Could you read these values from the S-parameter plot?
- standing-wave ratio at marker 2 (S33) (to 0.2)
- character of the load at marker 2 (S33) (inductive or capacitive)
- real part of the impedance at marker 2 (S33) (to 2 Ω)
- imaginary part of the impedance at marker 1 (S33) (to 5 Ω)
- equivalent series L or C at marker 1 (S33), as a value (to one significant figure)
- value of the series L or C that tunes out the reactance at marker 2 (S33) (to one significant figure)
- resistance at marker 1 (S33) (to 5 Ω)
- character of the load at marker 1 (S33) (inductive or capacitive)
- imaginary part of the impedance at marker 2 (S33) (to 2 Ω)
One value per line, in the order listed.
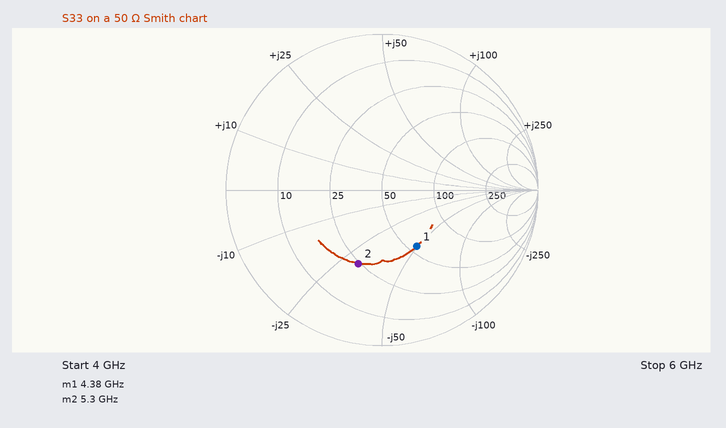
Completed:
3.0
capacitive
24 Ω
-50 Ω
700 fF
900 pH
55 Ω
capacitive
-30 Ω
